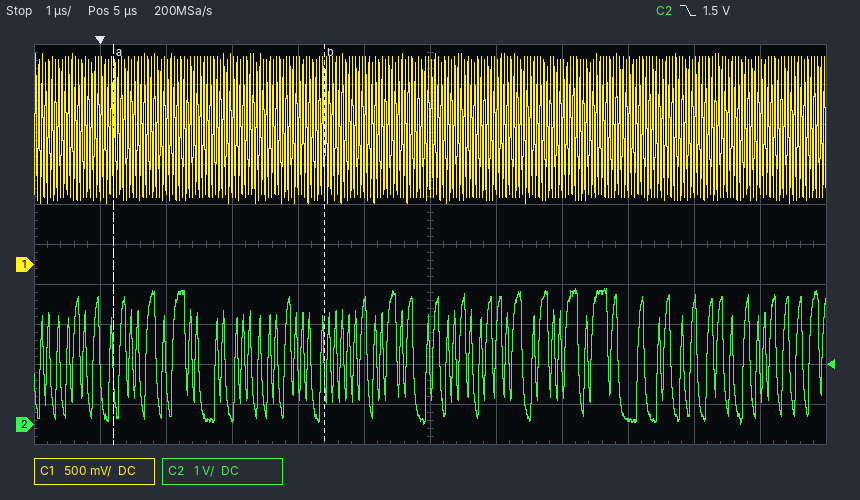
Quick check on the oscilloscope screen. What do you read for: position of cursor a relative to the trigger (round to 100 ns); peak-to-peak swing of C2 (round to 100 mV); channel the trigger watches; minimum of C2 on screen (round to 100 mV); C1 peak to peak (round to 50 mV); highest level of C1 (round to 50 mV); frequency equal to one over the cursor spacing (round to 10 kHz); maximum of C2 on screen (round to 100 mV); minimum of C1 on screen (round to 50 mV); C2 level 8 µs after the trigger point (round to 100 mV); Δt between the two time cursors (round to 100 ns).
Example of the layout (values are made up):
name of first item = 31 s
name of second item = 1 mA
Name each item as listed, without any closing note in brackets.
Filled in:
position of cursor a relative to the trigger = +200 ns
peak-to-peak swing of C2 = 3.4 V
channel the trigger watches = C2
minimum of C2 on screen = 0.0 V
C1 peak to peak = 1.90 V
highest level of C1 = 2.65 V
frequency equal to one over the cursor spacing = 310 kHz
maximum of C2 on screen = 3.4 V
minimum of C1 on screen = 750 mV
C2 level 8 µs after the trigger point = 100 mV
Δt between the two time cursors = 3.2 µs
